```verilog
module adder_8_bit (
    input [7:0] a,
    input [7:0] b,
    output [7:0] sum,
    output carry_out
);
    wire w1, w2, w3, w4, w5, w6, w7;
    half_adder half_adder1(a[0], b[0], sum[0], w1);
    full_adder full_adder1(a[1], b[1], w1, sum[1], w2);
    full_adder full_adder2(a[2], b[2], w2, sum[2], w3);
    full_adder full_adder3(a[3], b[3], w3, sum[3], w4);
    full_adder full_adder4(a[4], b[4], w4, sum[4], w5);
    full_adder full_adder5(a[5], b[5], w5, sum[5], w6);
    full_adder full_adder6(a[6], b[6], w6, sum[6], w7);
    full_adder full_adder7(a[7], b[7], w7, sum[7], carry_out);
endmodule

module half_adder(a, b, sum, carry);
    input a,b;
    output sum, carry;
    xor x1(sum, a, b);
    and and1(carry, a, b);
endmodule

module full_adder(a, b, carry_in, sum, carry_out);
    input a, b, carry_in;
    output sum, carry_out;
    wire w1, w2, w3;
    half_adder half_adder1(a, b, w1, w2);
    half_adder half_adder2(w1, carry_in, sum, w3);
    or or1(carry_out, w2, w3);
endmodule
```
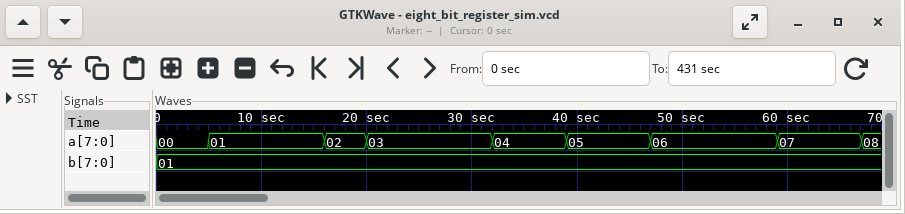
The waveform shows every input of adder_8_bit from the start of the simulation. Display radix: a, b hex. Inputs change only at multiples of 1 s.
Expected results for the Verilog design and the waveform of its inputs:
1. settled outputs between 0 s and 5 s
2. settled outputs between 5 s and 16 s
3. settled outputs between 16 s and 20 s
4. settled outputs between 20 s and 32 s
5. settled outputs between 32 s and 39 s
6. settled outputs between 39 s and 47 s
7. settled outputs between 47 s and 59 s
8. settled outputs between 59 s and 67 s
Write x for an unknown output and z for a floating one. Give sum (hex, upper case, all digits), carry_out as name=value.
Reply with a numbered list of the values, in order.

1. sum=01, carry_out=0
2. sum=02, carry_out=0
3. sum=03, carry_out=0
4. sum=04, carry_out=0
5. sum=05, carry_out=0
6. sum=06, carry_out=0
7. sum=07, carry_out=0
8. sum=08, carry_out=0
